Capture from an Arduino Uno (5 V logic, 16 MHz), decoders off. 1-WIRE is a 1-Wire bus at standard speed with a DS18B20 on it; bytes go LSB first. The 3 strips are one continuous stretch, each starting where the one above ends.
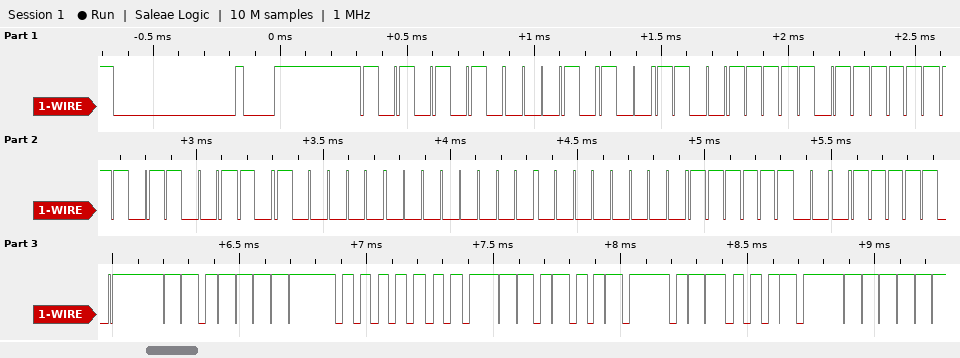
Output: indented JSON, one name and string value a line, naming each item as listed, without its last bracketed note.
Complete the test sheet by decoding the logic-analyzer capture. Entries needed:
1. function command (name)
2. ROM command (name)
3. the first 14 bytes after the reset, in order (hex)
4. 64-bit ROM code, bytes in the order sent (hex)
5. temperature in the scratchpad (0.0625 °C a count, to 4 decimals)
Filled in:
{
  "function command": "Read Scratchpad",
  "ROM command": "Match ROM",
  "the first 14 bytes after the reset, in order": "55 28 F3 FD 9B 05 00 00 3F BE FB 00 4B 46",
  "64-bit ROM code, bytes in the order sent": "28 F3 FD 9B 05 00 00 3F",
  "temperature in the scratchpad": "15.6875 °C"
}
